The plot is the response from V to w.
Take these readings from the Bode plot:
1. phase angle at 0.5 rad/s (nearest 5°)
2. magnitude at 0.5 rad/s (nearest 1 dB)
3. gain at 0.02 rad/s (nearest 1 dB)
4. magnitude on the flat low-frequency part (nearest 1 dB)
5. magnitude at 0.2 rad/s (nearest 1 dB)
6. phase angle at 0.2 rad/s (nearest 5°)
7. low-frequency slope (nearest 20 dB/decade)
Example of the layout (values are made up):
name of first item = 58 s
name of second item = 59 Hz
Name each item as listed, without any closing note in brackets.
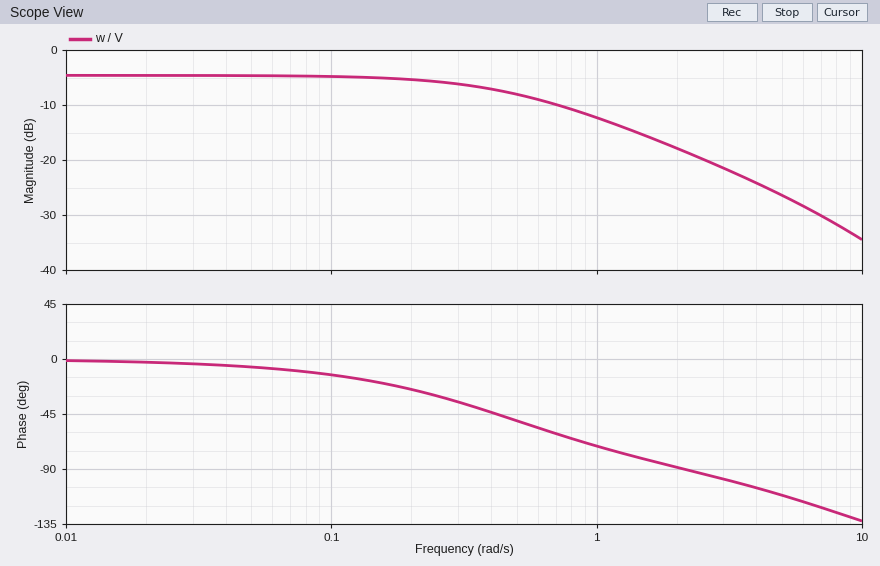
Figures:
phase angle at 0.5 rad/s = -50°
magnitude at 0.5 rad/s = -8 dB
gain at 0.02 rad/s = -5 dB
magnitude on the flat low-frequency part = -5 dB
magnitude at 0.2 rad/s = -5 dB
phase angle at 0.2 rad/s = -25°
low-frequency slope = 0 dB/decade
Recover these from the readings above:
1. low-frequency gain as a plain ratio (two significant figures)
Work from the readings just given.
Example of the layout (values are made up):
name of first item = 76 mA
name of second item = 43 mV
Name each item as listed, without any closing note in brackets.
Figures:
low-frequency gain as a plain ratio = 0.56
